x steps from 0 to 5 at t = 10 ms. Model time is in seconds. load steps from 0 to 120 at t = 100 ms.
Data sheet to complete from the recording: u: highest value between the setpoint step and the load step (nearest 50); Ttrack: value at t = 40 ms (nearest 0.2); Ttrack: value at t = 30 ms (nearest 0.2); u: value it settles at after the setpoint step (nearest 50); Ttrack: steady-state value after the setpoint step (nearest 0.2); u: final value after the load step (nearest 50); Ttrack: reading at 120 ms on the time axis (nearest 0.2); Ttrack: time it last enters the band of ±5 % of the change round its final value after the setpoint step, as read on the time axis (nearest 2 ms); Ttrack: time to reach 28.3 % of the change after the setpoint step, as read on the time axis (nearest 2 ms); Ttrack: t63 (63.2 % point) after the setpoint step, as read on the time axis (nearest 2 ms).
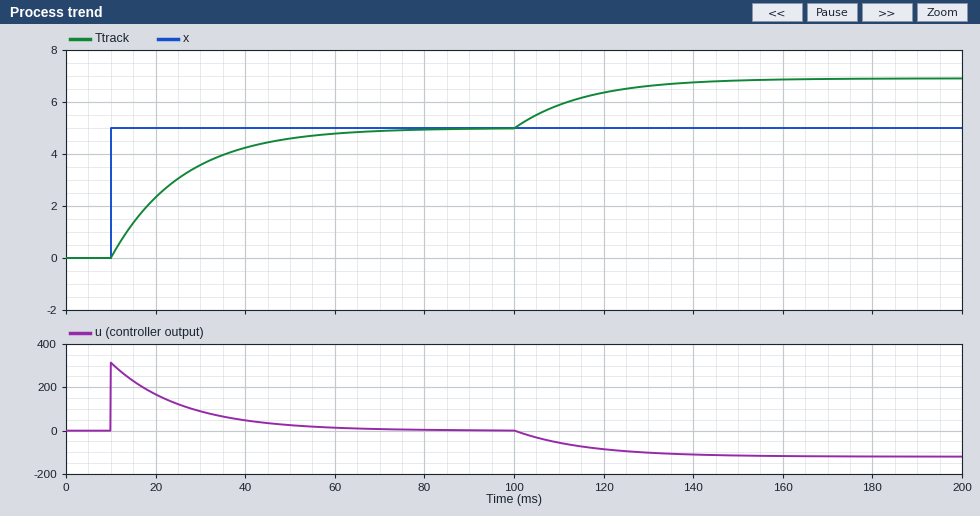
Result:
300
4.2
3.6
0
5.0
-100
6.4
58 ms
16 ms
26 ms
